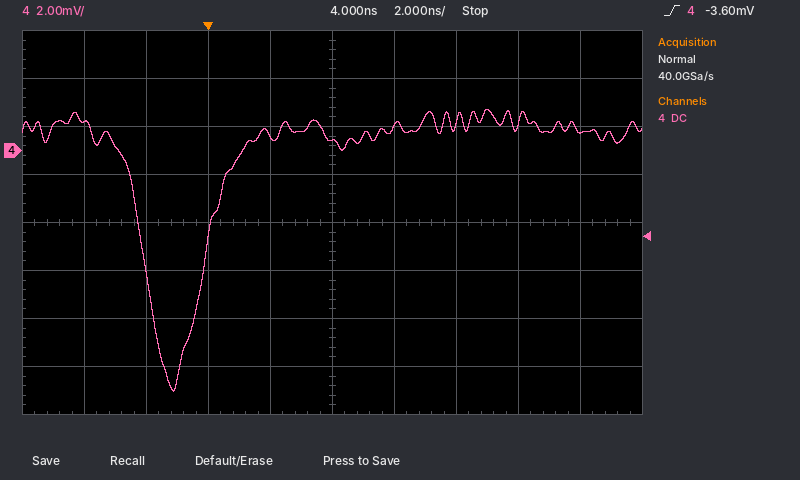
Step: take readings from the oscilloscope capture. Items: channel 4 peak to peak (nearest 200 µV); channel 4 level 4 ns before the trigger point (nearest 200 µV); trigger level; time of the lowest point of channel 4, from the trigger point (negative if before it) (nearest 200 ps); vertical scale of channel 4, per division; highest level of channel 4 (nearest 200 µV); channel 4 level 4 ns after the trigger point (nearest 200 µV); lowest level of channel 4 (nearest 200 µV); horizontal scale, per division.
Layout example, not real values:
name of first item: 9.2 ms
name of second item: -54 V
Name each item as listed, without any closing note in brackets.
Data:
channel 4 peak to peak: 11.8 mV
channel 4 level 4 ns before the trigger point: 1.2 mV
trigger level: -3.60 mV
time of the lowest point of channel 4, from the trigger point (negative if before it): -1.2 ns
vertical scale of channel 4, per division: 2 mV
highest level of channel 4: 1.8 mV
channel 4 level 4 ns after the trigger point: 400 µV
lowest level of channel 4: -10.0 mV
horizontal scale, per division: 2 ns
